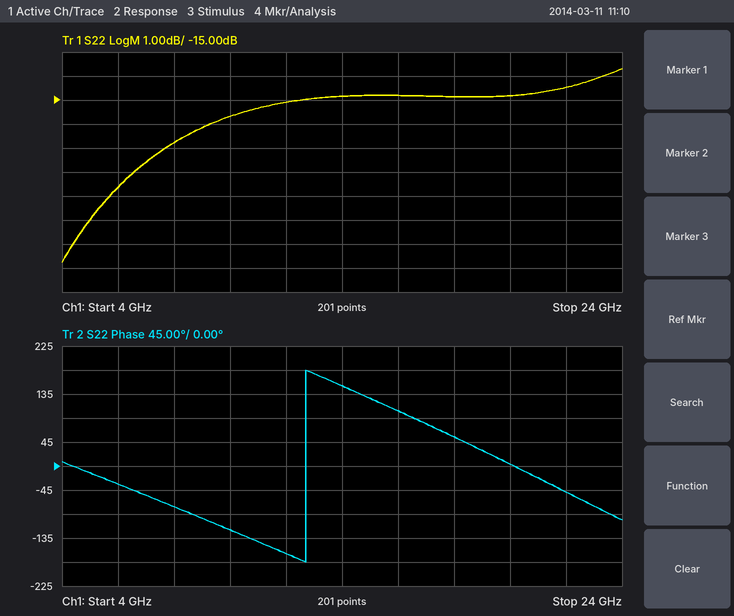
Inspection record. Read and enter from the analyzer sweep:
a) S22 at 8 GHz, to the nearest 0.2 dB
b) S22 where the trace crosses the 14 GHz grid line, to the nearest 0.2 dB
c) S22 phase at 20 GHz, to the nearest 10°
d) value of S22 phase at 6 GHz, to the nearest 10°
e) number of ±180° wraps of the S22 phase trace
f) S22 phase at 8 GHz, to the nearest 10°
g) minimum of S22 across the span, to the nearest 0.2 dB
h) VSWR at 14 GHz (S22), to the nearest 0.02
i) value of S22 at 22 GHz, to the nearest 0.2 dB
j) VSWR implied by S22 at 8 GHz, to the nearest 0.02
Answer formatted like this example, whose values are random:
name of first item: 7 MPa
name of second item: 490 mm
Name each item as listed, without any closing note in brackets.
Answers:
S22 at 8 GHz, to the nearest 0.2 dB: -16.8 dB
S22 where the trace crosses the 14 GHz grid line, to the nearest 0.2 dB: -14.8 dB
S22 phase at 20 GHz, to the nearest 10°: 0°
value of S22 phase at 6 GHz, to the nearest 10°: -30°
number of ±180° wraps of the S22 phase trace: 1
S22 phase at 8 GHz, to the nearest 10°: -80°
minimum of S22 across the span, to the nearest 0.2 dB: -21.8 dB
VSWR at 14 GHz (S22), to the nearest 0.02: 1.44
value of S22 at 22 GHz, to the nearest 0.2 dB: -14.4 dB
VSWR implied by S22 at 8 GHz, to the nearest 0.02: 1.34
